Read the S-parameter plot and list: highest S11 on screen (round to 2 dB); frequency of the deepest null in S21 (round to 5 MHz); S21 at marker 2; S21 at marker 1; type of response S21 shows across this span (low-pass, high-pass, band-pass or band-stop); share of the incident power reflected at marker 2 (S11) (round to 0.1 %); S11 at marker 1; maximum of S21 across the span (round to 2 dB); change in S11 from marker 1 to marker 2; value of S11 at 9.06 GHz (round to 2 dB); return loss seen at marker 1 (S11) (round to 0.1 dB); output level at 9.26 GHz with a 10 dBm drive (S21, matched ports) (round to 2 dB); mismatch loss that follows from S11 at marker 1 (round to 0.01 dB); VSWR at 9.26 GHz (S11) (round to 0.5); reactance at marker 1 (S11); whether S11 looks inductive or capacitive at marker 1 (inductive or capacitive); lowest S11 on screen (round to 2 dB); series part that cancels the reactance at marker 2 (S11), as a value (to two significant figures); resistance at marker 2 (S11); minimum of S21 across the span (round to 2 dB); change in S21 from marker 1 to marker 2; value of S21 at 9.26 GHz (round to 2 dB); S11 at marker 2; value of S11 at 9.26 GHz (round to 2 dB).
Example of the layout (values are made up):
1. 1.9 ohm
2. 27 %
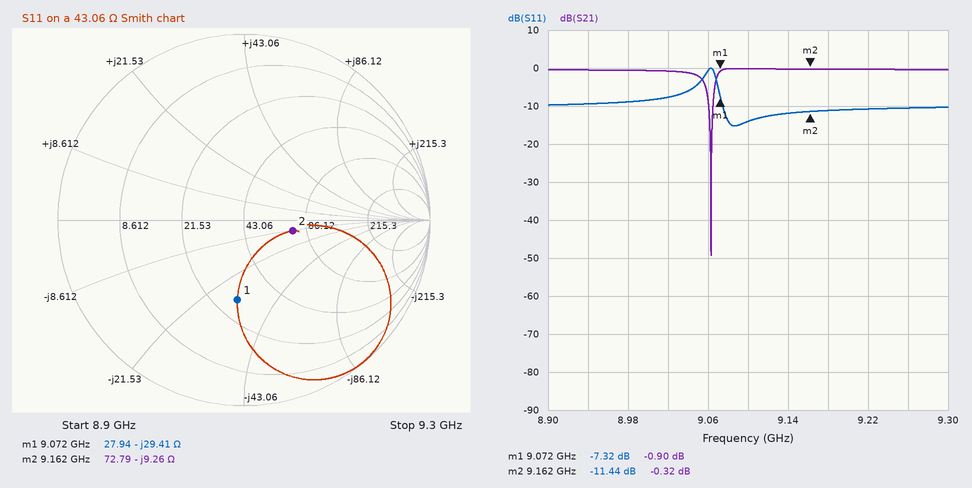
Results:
1. 0 dB
2. 9.065 GHz
3. -0.32 dB
4. -0.90 dB
5. band-stop
6. 7.2 %
7. -7.32 dB
8. 0 dB
9. -4.12 dB
10. 0 dB
11. 7.3 dB
12. 10 dBm
13. 0.89 dB
14. 2.0
15. -29.41 Ω
16. capacitive
17. -16 dB
18. 160 pH
19. 72.79 Ω
20. -50 dB
21. 0.58 dB
22. 0 dB
23. -11.44 dB
24. -10 dB
